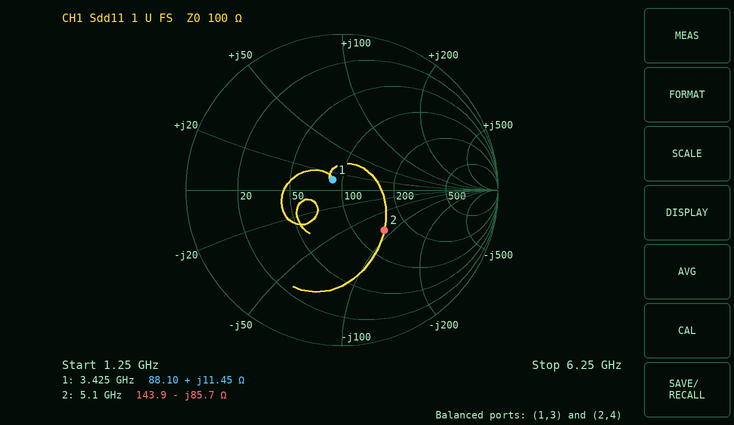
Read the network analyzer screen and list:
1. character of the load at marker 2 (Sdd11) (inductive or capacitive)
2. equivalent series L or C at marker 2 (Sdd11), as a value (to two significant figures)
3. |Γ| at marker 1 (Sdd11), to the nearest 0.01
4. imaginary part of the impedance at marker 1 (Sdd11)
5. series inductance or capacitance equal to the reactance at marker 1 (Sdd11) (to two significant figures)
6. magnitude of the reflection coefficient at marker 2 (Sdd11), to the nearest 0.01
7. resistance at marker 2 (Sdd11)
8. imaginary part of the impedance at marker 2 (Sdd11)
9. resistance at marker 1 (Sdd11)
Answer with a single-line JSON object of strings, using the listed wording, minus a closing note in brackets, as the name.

{"character of the load at marker 2 (Sdd11)": "capacitive", "equivalent series L or C at marker 2 (Sdd11), as a value": "360 fF", "|Γ| at marker 1 (Sdd11), to the nearest 0.01": "0.09", "imaginary part of the impedance at marker 1": "+11.45 Ω", "series inductance or capacitance equal to the reactance at marker 1 (Sdd11)": "530 pH", "magnitude of the reflection coefficient at marker 2 (Sdd11), to the nearest 0.01": "0.37", "resistance at marker 2": "143.9 Ω", "imaginary part of the impedance at marker 2": "-85.7 Ω", "resistance at marker 1": "88.10 Ω"}
